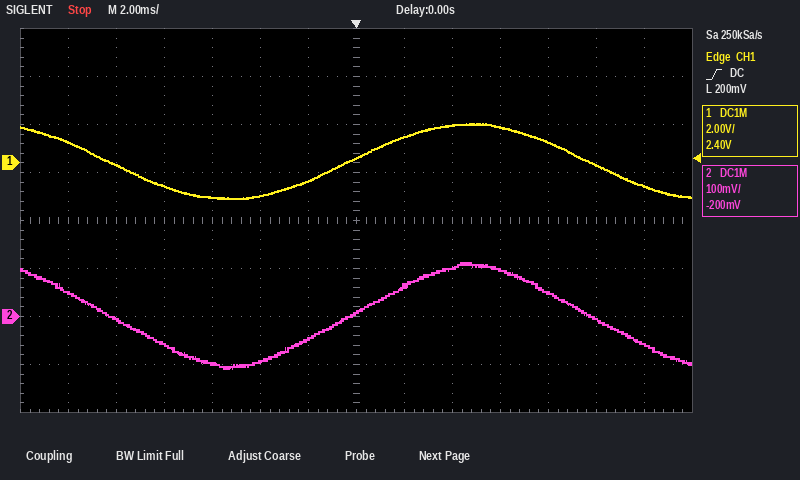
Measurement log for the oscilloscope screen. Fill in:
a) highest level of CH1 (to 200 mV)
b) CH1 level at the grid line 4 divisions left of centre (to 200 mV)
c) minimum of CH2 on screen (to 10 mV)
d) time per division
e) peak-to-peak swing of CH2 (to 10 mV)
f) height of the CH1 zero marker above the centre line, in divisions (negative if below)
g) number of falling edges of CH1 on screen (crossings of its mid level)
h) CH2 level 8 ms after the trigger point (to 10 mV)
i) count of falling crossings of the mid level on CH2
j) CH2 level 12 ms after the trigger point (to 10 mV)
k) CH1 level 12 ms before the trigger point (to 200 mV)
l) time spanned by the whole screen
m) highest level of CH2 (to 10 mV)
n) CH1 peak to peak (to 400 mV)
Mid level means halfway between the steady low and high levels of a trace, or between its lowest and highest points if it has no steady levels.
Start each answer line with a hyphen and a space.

- 1.6 V
- -1.0 V
- -110 mV
- 2 ms
- 220 mV
- +1.2 div
- 2
- 50 mV
- 2
- -60 mV
- 800 mV
- 28 ms
- 110 mV
- 3.2 V
